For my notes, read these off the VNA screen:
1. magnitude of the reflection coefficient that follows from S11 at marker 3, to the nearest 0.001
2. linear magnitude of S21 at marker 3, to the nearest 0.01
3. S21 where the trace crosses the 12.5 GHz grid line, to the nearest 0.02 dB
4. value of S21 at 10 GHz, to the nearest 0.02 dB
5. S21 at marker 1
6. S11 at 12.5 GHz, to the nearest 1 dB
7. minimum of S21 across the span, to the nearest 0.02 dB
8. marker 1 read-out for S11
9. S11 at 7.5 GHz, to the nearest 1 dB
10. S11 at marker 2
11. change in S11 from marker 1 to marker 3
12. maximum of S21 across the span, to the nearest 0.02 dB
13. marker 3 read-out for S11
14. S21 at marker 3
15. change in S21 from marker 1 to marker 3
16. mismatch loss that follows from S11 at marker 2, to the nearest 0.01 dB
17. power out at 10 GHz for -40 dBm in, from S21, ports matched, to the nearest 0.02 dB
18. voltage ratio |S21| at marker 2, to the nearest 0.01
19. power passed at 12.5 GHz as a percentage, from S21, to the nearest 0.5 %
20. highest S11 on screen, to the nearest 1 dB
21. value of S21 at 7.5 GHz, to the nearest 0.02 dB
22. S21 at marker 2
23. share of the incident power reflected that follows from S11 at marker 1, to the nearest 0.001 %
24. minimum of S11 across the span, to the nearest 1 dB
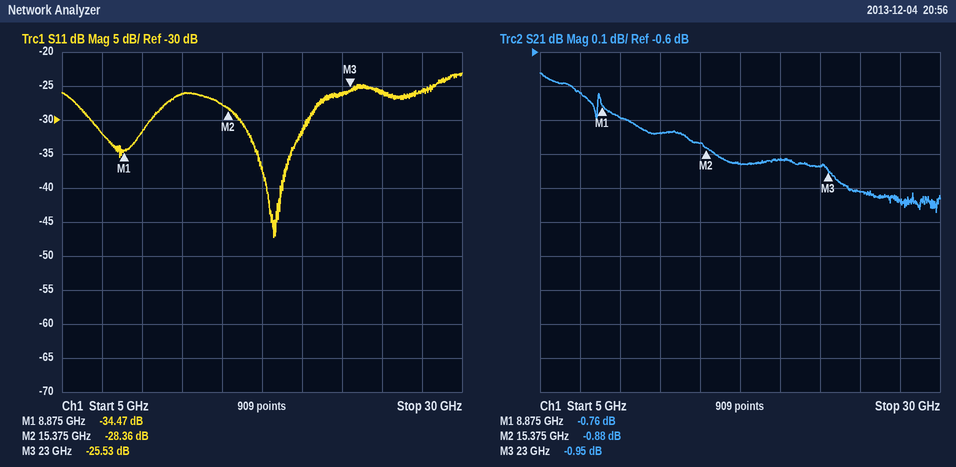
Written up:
0.053
0.90
-0.84 dB
-0.80 dB
-0.76 dB
-26 dB
-1.08 dB
-34.47 dB
-32 dB
-28.36 dB
8.94 dB
-0.66 dB
-25.53 dB
-0.95 dB
-0.19 dB
0.01 dB
-40.80 dBm
0.90
82.5 %
-23 dB
-0.72 dB
-0.88 dB
0.036 %
-47 dB
